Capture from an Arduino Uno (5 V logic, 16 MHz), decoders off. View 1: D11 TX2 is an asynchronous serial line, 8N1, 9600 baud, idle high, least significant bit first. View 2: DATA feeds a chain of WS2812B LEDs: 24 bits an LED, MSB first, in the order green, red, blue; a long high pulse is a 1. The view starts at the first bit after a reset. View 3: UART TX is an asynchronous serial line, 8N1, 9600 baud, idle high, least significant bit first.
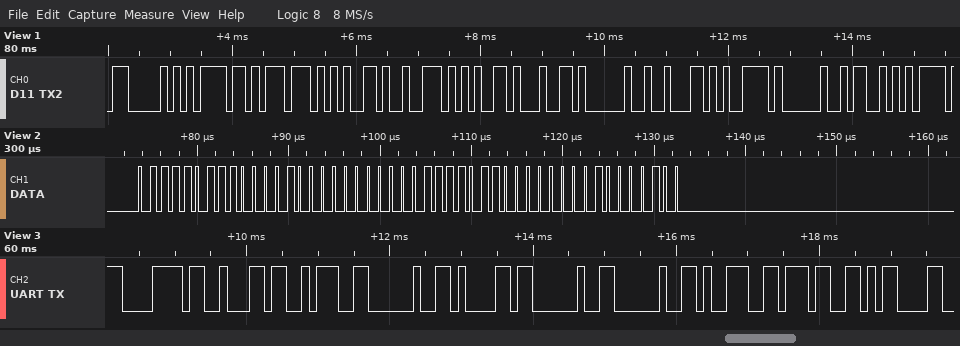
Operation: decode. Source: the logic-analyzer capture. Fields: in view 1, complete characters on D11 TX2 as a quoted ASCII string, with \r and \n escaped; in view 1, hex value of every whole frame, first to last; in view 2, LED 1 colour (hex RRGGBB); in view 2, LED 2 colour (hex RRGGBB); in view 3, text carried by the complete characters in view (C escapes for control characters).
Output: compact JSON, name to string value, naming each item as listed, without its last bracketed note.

{"in view 1, complete characters on D11 TX2 as a quoted ASCII string, with \\r and \\n escaped": "\"Powered by S\"", "in view 1, hex value of every whole frame, first to last": "50 6F 77 65 72 65 64 20 62 79 20 53", "in view 2, LED 1 colour": "#847B00", "in view 2, LED 2 colour": "#007B84", "in view 3, text carried by the complete characters in view": "\"xb: a  97\\r\""}
